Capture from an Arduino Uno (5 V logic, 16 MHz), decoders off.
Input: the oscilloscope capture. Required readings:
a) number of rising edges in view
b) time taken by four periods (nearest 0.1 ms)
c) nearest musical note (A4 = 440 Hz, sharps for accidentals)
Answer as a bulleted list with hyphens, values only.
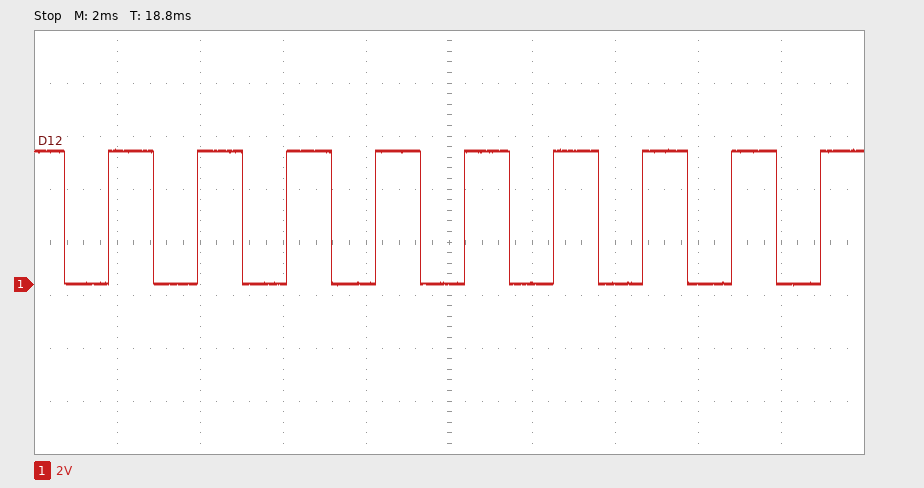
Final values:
- 9
- 8.6 ms
- A#4
